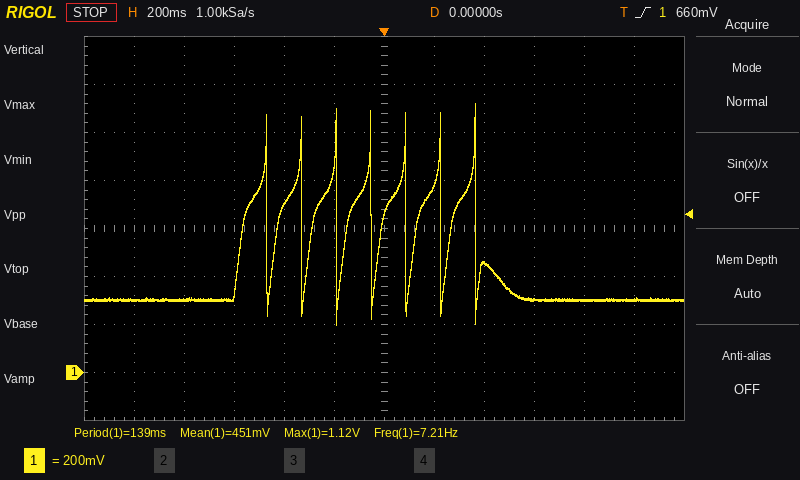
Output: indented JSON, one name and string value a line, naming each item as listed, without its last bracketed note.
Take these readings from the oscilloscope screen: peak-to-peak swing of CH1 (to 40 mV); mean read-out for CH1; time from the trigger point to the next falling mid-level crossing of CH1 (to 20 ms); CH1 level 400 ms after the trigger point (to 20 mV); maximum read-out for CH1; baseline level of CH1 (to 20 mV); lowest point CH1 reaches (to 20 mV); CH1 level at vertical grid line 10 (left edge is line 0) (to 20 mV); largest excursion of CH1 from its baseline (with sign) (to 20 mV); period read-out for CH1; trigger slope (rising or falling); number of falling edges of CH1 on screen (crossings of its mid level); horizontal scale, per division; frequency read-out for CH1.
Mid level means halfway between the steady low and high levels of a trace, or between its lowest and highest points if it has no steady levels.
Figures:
{
  "peak-to-peak swing of CH1": "920 mV",
  "mean read-out for CH1": "451 mV",
  "time from the trigger point to the next falling mid-level crossing of CH1": "80 ms",
  "CH1 level 400 ms after the trigger point": "460 mV",
  "maximum read-out for CH1": "1.12 V",
  "baseline level of CH1": "300 mV",
  "lowest point CH1 reaches": "200 mV",
  "CH1 level at vertical grid line 10 (left edge is line 0)": "300 mV",
  "largest excursion of CH1 from its baseline (with sign)": "+820 mV",
  "period read-out for CH1": "139 ms",
  "trigger slope": "rising",
  "number of falling edges of CH1 on screen": "7",
  "horizontal scale, per division": "200 ms",
  "frequency read-out for CH1": "7.21 Hz"
}
